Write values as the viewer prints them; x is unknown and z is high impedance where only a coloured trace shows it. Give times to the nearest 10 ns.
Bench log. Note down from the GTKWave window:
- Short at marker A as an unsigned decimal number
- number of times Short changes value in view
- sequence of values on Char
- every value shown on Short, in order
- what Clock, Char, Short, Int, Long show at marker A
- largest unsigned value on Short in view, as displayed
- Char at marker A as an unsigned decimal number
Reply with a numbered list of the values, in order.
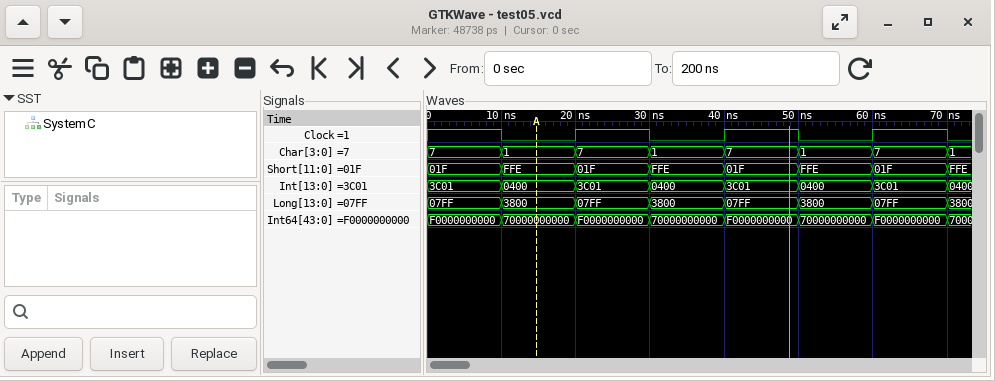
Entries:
1. 4094
2. 7
3. 7, 1, 7, 1, 7, 1, 7, 1
4. 01F, FFE, 01F, FFE, 01F, FFE, 01F, FFE
5. Clock=0, Char=1, Short=FFE, Int=0400, Long=3800
6. FFE
7. 1
